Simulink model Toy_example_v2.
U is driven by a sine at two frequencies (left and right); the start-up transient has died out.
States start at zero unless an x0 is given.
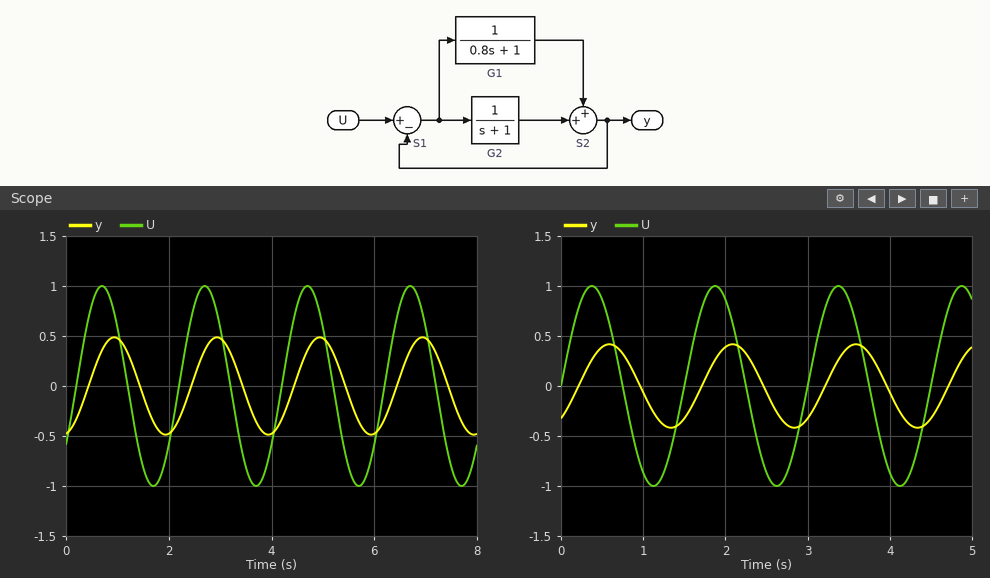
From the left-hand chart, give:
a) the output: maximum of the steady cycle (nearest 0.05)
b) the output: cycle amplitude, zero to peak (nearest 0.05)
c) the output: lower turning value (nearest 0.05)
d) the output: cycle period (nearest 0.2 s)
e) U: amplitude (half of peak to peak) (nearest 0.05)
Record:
0.50
0.50
-0.50
2.0 s
1.00
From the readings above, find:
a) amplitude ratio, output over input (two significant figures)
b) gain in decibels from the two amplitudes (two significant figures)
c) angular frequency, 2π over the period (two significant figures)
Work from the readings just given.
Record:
0.50
-6.0 dB
3.1 rad/s
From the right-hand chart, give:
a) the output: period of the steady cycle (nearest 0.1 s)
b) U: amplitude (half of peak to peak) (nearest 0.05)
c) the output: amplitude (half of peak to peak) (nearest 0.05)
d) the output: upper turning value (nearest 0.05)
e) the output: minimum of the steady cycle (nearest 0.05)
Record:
1.5 s
1.00
0.40
0.40
-0.40
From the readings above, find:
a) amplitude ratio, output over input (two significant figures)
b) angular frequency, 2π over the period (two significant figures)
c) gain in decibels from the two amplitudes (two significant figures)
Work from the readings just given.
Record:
0.40
4.2 rad/s
-8.0 dB
